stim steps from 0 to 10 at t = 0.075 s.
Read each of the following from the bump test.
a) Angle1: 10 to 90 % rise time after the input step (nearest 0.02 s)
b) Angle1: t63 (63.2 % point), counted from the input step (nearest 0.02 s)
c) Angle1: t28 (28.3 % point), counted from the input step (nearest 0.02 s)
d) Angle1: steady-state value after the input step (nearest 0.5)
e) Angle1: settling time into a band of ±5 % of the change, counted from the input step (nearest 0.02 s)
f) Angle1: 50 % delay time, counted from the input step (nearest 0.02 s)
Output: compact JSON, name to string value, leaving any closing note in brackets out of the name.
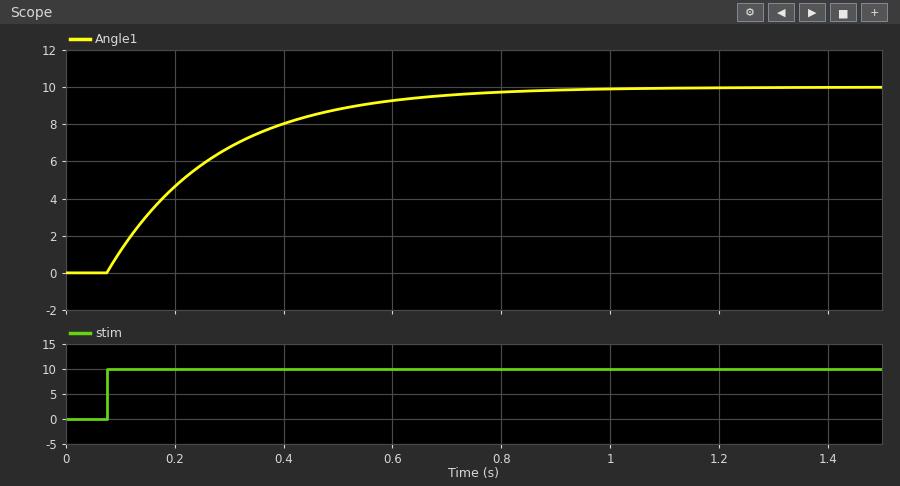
{"Angle1: 10 to 90 % rise time after the input step": "0.44 s", "Angle1: t63 (63.2 % point), counted from the input step": "0.20 s", "Angle1: t28 (28.3 % point), counted from the input step": "0.06 s", "Angle1: steady-state value after the input step": "10.0", "Angle1: settling time into a band of ±5 % of the change, counted from the input step": "0.60 s", "Angle1: 50 % delay time, counted from the input step": "0.14 s"}
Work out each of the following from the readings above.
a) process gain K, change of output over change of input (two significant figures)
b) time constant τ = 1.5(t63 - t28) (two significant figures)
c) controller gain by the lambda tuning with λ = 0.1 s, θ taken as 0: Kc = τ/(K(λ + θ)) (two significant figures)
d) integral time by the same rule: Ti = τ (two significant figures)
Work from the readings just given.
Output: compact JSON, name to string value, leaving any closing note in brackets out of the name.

{"process gain K, change of output over change of input": "1.0", "time constant τ = 1.5(t63 - t28)": "0.21 s", "controller gain by the lambda tuning with λ = 0.1 s, θ taken as 0: Kc = τ/(K(λ + θ))": "2.1", "integral time by the same rule: Ti = τ": "0.21 s"}
